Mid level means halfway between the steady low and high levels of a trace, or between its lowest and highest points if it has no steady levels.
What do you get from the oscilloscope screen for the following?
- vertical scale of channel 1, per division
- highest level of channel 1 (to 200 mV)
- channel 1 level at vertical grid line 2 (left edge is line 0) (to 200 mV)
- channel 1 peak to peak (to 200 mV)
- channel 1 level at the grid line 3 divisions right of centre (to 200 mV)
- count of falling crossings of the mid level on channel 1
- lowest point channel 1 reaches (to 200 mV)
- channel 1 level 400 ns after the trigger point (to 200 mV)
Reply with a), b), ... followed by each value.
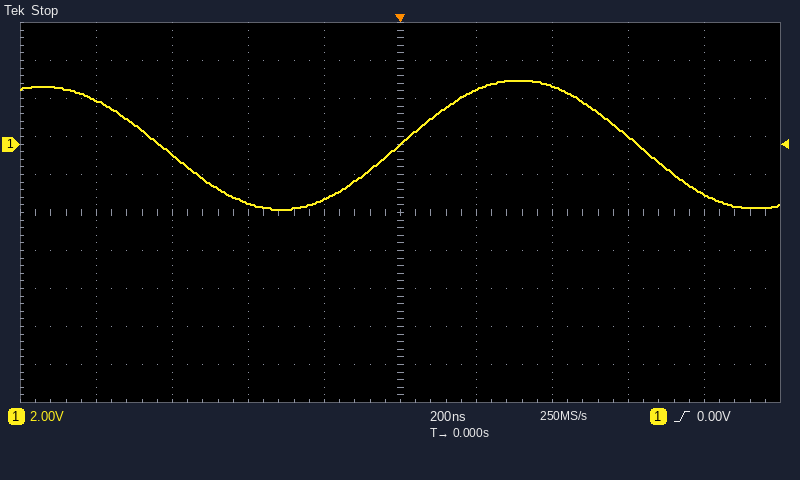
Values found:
a) 2 V
b) 3.4 V
c) -600 mV
d) 6.8 V
e) 400 mV
f) 2
g) -3.4 V
h) 3.0 V
